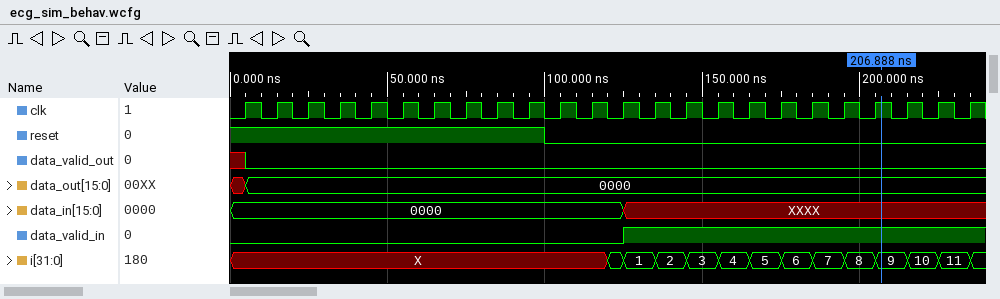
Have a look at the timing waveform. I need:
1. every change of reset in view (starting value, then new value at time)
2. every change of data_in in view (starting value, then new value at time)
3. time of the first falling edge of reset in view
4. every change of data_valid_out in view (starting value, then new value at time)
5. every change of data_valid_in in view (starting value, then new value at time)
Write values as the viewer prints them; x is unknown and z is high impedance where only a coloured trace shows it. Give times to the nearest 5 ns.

1, 0 at 100 ns
0000, XXXX at 125 ns
100 ns
x, 0 at 5 ns
0, 1 at 125 ns
